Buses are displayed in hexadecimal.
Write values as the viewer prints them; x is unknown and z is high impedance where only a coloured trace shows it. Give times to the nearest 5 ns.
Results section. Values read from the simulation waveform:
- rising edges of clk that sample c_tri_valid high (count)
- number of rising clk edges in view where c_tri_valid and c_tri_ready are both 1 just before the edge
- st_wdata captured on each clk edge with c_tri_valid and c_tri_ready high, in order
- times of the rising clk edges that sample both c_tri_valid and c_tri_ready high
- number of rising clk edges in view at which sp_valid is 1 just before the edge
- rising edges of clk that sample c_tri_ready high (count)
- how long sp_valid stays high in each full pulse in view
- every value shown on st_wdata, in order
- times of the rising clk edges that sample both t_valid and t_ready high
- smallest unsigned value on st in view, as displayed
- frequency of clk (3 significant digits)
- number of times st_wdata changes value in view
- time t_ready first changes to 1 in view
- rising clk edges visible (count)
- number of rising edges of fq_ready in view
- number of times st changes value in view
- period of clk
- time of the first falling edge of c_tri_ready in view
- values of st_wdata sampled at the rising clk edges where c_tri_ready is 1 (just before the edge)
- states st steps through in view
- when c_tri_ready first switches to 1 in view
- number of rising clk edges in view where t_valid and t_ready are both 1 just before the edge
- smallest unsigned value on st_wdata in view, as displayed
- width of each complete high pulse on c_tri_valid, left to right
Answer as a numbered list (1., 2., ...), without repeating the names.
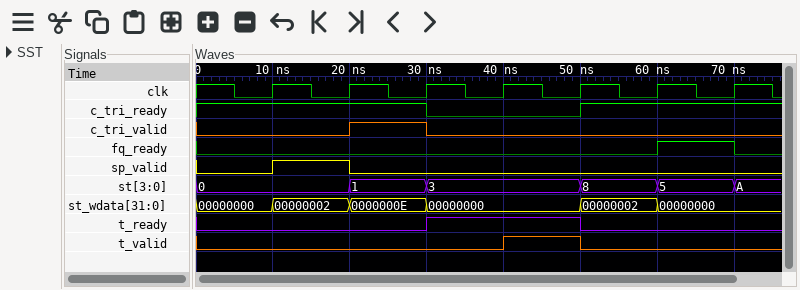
1. 1
2. 1
3. 0000000E
4. 30 ns
5. 1
6. 5
7. 10 ns
8. 00000000, 00000002, 0000000E, 00000000, 00000002, 00000000
9. 50 ns
10. 0
11. 100 MHz
12. 5
13. 30 ns
14. 7
15. 1
16. 5
17. 10 ns
18. 30 ns
19. 00000000, 00000002, 0000000E, 00000002, 00000000
20. 0, 1, 3, 8, 5, A
21. 50 ns
22. 1
23. 00000000
24. 10 ns
